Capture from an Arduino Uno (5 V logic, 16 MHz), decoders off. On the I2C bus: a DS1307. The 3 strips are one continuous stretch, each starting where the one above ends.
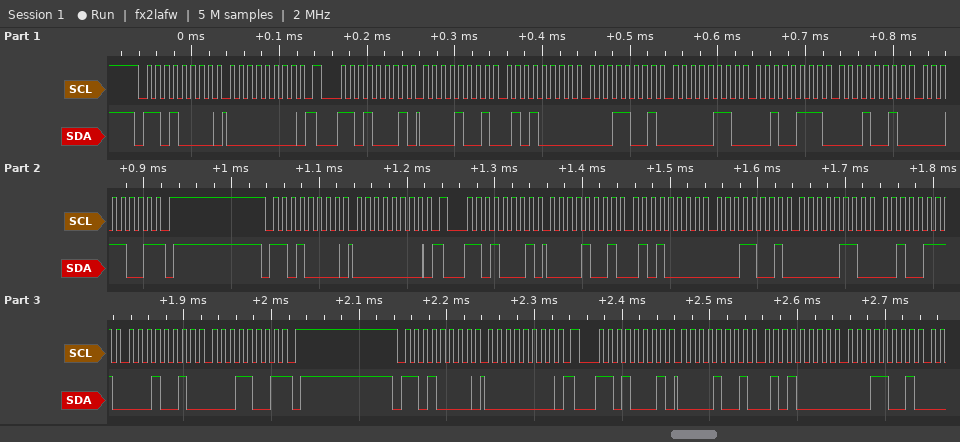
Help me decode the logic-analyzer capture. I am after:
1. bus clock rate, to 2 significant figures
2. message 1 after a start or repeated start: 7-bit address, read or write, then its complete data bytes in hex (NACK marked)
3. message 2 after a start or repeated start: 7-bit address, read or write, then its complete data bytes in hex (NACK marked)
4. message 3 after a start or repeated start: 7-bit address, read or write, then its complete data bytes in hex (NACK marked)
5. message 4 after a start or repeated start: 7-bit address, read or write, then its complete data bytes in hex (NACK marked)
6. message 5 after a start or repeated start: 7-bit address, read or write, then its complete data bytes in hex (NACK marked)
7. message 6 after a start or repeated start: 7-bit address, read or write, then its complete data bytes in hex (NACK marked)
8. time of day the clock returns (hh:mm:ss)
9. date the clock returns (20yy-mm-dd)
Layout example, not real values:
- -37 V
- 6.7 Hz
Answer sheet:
- 100 kHz
- 0x68 write: 00
- 0x68 read: 09 50 19 06 27 12 19 NACK
- 0x68 write: 00
- 0x68 read: 09 50 19 06 27 12 19 NACK
- 0x68 write: 00
- 0x68 read: 09 50 19
- 19:50:09
- 2019-12-27
